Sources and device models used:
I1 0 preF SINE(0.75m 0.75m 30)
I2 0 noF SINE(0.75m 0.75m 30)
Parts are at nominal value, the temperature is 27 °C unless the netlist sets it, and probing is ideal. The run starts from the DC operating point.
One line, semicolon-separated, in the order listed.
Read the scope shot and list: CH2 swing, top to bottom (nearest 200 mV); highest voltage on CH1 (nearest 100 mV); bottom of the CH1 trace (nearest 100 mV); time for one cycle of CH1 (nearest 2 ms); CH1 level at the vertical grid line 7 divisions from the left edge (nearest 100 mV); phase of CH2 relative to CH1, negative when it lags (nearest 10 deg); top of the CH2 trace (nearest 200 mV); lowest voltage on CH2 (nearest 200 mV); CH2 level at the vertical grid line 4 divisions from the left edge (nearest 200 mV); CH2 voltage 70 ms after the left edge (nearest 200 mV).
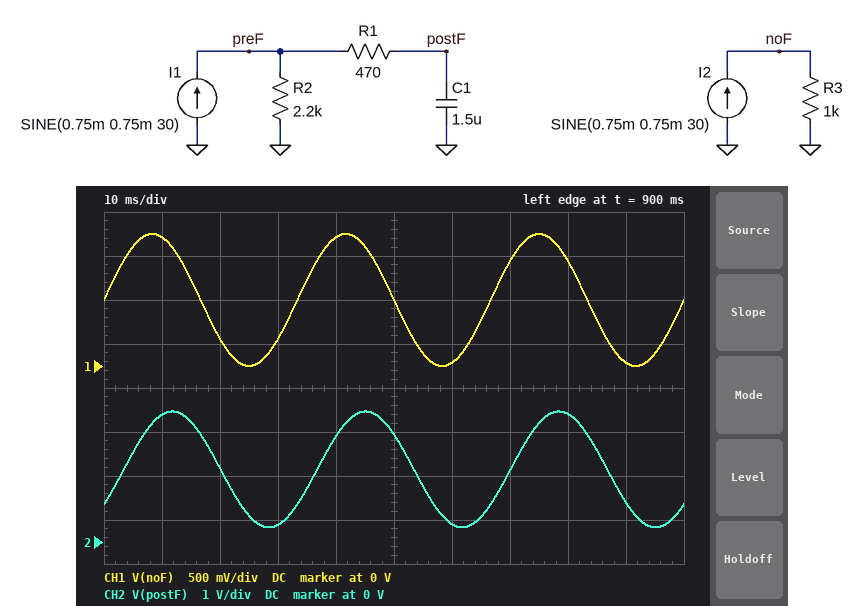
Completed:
2.6 V; 1.5 V; 0 V; 34 ms; 1.2 V; -40 deg; 3.0 V; 400 mV; 2.4 V; 1.6 V
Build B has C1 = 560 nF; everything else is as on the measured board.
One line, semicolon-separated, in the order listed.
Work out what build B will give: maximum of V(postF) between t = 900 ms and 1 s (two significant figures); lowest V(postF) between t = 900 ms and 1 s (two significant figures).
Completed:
3.2 V; 62 mV
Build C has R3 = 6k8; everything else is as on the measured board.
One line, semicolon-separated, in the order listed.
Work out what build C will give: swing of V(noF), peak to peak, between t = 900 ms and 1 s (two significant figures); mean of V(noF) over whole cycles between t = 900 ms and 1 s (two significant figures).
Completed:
10 V; 5.1 V
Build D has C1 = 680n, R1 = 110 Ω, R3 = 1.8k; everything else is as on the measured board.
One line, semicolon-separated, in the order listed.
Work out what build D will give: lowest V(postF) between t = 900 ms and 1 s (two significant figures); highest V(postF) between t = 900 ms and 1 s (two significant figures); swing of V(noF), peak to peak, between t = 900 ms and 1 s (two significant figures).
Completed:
68 mV; 3.2 V; 2.7 V
